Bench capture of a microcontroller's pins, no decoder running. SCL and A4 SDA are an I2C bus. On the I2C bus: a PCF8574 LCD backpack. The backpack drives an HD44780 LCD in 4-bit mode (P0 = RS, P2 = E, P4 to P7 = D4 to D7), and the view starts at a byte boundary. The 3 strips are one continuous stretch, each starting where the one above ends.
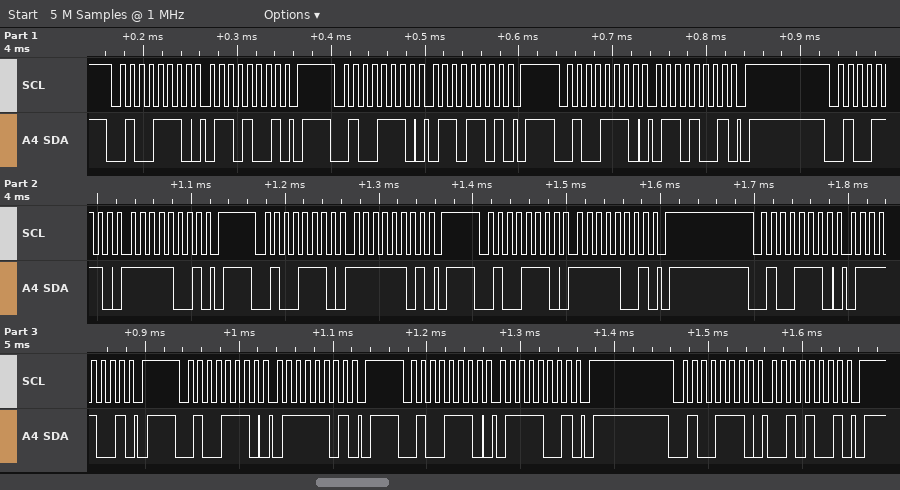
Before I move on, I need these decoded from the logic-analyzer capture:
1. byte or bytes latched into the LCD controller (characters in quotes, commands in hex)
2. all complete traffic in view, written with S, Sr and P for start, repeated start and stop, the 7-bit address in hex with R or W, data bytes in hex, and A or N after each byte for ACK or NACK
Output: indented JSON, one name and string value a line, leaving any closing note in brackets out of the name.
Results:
{
  "byte or bytes latched into the LCD controller": "'o'",
  "all complete traffic in view, written with S, Sr and P for start, repeated start and stop, the 7-bit address in hex with R or W, data bytes in hex, and A or N after each byte for ACK or NACK": "S 27W A 69 A P S 27W A 6D A P S 27W A 69 A P S 27W A F9 A P S 27W A FD A P S 27W A F9 A P S 27W A 79 A P S 27W A 7D A P S 27W A 79 A P S 27W A 29 A P"
}
